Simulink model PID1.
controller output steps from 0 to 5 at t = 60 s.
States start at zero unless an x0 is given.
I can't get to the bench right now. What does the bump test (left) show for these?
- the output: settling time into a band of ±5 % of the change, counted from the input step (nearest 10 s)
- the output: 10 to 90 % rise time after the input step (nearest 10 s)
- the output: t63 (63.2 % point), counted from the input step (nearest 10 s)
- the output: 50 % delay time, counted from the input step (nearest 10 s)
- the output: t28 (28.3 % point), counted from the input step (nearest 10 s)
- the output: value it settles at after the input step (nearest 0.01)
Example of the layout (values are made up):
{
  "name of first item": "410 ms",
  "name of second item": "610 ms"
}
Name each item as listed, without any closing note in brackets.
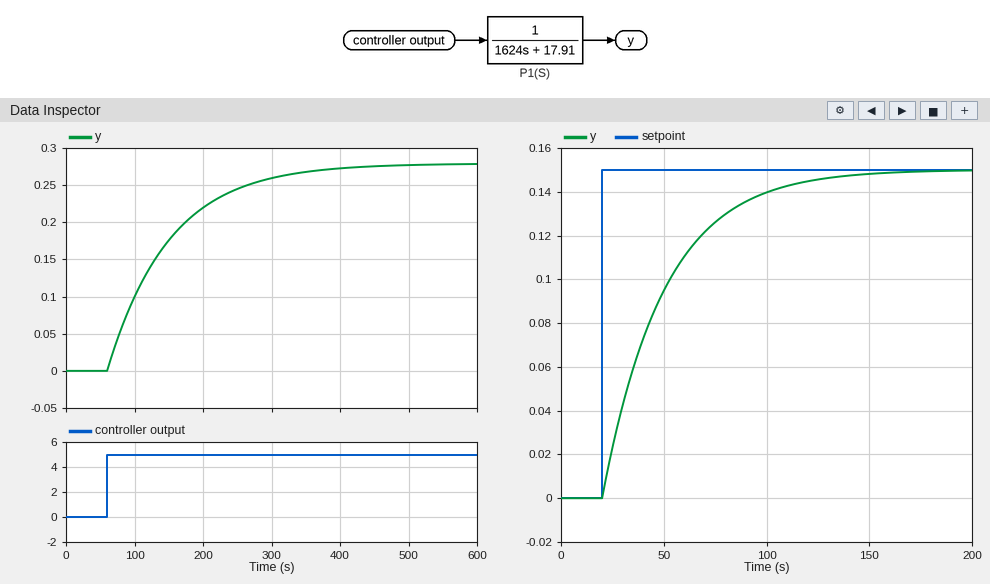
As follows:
{
  "the output: settling time into a band of ±5 % of the change, counted from the input step": "270 s",
  "the output: 10 to 90 % rise time after the input step": "200 s",
  "the output: t63 (63.2 % point), counted from the input step": "90 s",
  "the output: 50 % delay time, counted from the input step": "60 s",
  "the output: t28 (28.3 % point), counted from the input step": "30 s",
  "the output: value it settles at after the input step": "0.28"
}
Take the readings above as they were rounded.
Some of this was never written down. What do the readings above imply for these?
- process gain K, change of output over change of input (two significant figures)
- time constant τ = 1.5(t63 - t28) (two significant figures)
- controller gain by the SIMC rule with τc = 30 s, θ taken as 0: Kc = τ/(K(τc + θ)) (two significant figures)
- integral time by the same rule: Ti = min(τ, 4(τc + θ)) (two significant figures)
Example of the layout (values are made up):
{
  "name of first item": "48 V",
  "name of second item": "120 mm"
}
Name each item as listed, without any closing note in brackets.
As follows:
{
  "process gain K, change of output over change of input": "0.056",
  "time constant τ = 1.5(t63 - t28)": "90 s",
  "controller gain by the SIMC rule with τc = 30 s, θ taken as 0: Kc = τ/(K(τc + θ))": "54",
  "integral time by the same rule: Ti = min(τ, 4(τc + θ))": "90 s"
}
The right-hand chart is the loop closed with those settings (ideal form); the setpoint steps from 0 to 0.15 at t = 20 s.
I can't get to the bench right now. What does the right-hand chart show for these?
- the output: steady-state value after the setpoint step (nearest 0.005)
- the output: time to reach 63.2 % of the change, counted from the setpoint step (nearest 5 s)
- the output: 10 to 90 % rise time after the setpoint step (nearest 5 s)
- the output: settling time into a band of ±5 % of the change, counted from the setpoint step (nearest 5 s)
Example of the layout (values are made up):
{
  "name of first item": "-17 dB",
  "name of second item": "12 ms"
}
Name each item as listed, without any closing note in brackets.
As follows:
{
  "the output: steady-state value after the setpoint step": "0.150",
  "the output: time to reach 63.2 % of the change, counted from the setpoint step": "30 s",
  "the output: 10 to 90 % rise time after the setpoint step": "65 s",
  "the output: settling time into a band of ±5 % of the change, counted from the setpoint step": "90 s"
}
